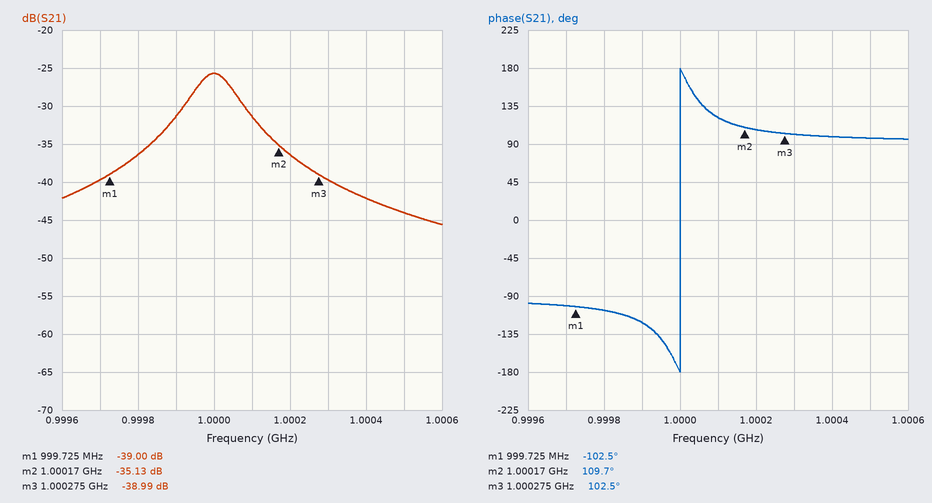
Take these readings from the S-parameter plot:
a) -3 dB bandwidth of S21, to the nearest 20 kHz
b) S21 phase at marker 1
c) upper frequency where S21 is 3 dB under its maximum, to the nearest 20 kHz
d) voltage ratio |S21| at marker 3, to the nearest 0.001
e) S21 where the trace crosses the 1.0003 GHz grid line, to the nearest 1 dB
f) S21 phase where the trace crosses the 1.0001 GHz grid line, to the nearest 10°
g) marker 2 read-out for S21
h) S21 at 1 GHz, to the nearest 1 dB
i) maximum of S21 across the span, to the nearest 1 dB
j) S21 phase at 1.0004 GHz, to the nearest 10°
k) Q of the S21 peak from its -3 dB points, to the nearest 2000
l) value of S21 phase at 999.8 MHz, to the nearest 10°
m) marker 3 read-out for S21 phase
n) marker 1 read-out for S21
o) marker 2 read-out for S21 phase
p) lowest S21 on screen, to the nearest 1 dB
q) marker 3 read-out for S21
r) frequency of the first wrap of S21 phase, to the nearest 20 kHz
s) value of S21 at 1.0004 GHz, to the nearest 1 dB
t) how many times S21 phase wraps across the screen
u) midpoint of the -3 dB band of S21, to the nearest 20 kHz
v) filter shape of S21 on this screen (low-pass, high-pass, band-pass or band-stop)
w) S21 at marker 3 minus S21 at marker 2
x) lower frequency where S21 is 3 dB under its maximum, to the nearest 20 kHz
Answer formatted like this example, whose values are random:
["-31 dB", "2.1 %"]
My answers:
["120 kHz", "-102.5°", "1.00006 GHz", "0.011", "-40 dB", "120°", "-35.13 dB", "-26 dB", "-26 dB", "100°", "8000", "-110°", "102.5°", "-39.00 dB", "109.7°", "-46 dB", "-38.99 dB", "1.00000 GHz", "-42 dB", "1", "1.00000 GHz", "band-pass", "-3.86 dB", "999.94 MHz"]
